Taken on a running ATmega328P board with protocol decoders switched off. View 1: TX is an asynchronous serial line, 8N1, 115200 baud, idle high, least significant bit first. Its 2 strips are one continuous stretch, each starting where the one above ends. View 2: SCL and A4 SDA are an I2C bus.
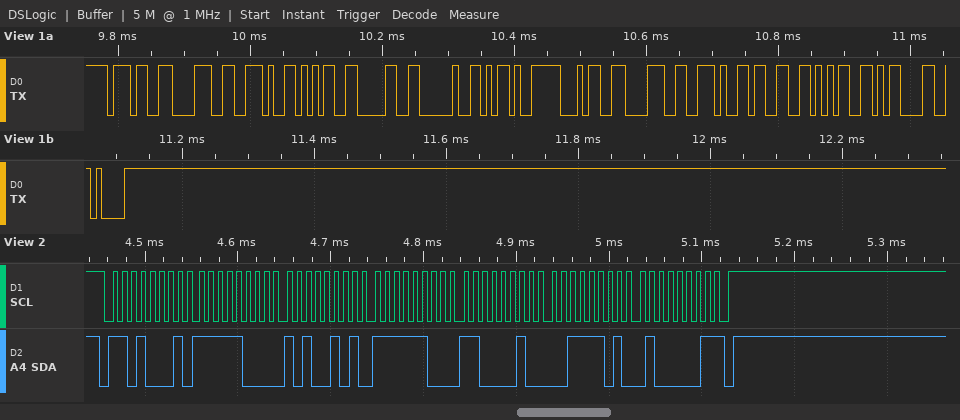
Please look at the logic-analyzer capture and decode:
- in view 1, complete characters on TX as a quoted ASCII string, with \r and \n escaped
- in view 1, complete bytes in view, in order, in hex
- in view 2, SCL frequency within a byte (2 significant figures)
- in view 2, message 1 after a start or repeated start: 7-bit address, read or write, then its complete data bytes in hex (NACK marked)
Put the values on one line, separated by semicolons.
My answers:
"78.50 -48.35\r\n"; 37 38 2E 35 30 20 2D 34 38 2E 33 35 0D 0A; 100 kHz; 0x68 read: F8 A5 FC C2 3D 41 NACK
